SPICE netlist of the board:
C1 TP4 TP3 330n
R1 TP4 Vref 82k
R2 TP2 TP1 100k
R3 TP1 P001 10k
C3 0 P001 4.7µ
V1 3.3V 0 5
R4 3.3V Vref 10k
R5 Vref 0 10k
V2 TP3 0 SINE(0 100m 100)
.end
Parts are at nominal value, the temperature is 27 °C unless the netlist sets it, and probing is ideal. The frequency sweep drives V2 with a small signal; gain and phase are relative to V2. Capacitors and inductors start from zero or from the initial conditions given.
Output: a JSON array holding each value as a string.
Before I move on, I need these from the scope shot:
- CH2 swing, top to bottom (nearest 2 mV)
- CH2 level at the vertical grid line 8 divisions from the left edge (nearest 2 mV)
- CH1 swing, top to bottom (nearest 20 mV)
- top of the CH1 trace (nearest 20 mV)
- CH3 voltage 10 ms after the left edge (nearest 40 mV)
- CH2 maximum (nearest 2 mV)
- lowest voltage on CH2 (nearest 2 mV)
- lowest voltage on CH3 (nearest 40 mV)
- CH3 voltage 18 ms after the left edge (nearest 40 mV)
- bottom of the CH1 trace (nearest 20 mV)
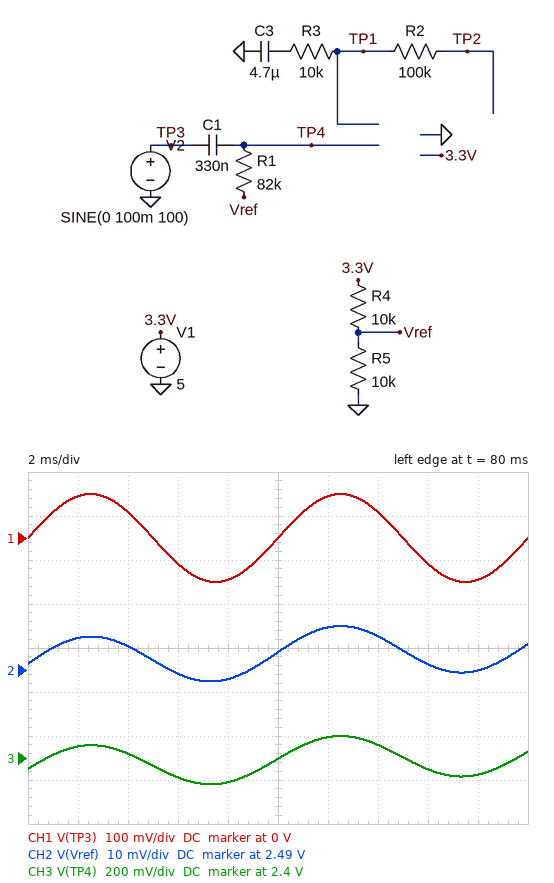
["12 mV", "2.492 V", "200 mV", "100 mV", "2.40 V", "2.500 V", "2.488 V", "2.28 V", "2.32 V", "-100 mV"]
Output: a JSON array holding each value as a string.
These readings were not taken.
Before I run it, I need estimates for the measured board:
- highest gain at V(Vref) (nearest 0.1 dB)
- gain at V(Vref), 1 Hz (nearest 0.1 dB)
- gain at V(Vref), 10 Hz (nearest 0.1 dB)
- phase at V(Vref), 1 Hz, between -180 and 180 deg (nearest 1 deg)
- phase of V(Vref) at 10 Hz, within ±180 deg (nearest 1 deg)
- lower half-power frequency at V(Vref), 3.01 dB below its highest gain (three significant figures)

["-24.8 dB", "-39.8 dB", "-26.0 dB", "80 deg", "29 deg", "5.54 Hz"]
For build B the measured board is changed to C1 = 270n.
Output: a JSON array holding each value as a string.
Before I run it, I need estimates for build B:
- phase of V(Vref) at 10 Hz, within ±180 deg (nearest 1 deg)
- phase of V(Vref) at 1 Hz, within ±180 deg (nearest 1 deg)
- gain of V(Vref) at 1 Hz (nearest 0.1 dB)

["34 deg", "82 deg", "-41.5 dB"]
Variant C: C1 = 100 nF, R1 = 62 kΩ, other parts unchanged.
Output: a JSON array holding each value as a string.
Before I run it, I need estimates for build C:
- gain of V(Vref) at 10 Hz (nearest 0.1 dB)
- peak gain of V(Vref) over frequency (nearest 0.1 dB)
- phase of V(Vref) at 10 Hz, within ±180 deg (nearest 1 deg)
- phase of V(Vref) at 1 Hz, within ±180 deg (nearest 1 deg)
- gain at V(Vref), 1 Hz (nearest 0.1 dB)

["-30.8 dB", "-22.5 dB", "67 deg", "88 deg", "-50.1 dB"]
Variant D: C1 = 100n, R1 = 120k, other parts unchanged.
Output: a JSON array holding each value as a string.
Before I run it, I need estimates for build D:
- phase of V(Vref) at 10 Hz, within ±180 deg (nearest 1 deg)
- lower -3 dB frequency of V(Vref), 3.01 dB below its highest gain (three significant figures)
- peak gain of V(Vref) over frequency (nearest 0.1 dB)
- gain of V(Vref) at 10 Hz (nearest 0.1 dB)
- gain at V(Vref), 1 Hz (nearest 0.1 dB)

["52 deg", "12.7 Hz", "-28.0 dB", "-32.1 dB", "-50.1 dB"]
